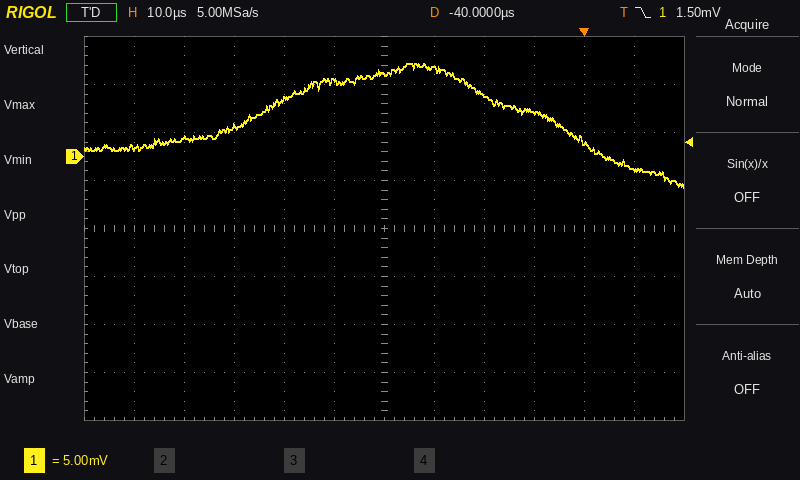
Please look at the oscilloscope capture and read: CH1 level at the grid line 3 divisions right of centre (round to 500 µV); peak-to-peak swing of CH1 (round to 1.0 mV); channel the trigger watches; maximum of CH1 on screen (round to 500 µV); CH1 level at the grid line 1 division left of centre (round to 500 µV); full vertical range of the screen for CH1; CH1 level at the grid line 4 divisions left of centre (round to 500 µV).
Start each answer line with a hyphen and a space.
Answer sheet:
- 4.5 mV
- 13.0 mV
- CH1
- 9.5 mV
- 8.0 mV
- 40 mV
- 2.0 mV
